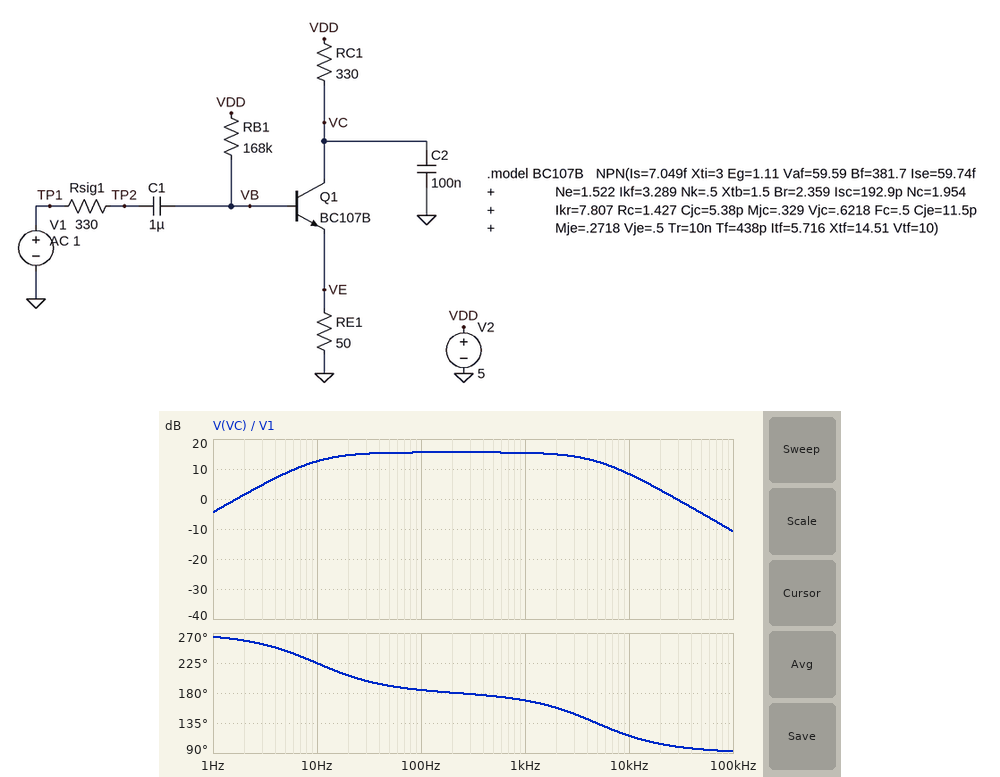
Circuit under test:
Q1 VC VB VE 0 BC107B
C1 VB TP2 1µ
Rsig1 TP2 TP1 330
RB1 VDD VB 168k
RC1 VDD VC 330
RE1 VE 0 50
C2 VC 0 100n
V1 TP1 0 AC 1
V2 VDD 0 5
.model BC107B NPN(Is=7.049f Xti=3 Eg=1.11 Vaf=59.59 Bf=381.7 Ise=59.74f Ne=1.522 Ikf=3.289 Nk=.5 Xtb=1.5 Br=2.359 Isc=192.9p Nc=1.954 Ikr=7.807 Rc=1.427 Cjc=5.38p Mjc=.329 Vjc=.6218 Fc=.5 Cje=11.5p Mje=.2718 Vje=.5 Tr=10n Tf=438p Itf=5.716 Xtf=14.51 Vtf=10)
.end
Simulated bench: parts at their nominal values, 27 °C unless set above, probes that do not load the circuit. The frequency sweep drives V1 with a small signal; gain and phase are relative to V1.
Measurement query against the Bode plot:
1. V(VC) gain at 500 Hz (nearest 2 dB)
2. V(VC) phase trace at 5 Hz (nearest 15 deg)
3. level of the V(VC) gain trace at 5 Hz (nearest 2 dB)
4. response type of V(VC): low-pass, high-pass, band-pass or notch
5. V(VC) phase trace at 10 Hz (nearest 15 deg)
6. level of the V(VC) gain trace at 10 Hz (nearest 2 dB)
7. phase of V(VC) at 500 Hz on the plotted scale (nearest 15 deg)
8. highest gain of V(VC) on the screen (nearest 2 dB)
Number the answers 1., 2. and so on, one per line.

1. 16 dB
2. 240 deg
3. 8 dB
4. band-pass
5. 225 deg
6. 12 dB
7. 180 deg
8. 16 dB
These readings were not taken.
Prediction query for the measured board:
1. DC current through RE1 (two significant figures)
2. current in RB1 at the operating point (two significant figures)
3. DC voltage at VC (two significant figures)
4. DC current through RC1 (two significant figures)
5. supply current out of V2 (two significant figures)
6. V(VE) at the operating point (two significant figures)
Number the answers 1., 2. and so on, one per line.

1. 7.3 mA
2. 23 µA
3. 2.6 V
4. 7.3 mA
5. 7.3 mA
6. 370 mV
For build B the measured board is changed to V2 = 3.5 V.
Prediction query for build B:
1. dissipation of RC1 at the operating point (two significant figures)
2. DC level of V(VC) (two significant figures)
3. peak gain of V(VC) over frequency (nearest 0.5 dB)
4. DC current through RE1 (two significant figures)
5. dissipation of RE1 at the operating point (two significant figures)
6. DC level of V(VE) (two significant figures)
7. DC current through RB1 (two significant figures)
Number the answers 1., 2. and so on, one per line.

1. 7.0 mW
2. 2.0 V
3. 15.0 dB
4. 4.6 mA
5. 1.1 mW
6. 230 mV
7. 15 µA
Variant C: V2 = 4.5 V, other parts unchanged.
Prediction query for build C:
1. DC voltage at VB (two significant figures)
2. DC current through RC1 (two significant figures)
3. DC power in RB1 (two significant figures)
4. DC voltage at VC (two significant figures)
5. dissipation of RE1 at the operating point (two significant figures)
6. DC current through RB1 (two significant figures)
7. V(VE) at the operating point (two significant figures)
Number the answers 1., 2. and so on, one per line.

1. 1.0 V
2. 6.4 mA
3. 72 µW
4. 2.4 V
5. 2.1 mW
6. 21 µA
7. 320 mV
